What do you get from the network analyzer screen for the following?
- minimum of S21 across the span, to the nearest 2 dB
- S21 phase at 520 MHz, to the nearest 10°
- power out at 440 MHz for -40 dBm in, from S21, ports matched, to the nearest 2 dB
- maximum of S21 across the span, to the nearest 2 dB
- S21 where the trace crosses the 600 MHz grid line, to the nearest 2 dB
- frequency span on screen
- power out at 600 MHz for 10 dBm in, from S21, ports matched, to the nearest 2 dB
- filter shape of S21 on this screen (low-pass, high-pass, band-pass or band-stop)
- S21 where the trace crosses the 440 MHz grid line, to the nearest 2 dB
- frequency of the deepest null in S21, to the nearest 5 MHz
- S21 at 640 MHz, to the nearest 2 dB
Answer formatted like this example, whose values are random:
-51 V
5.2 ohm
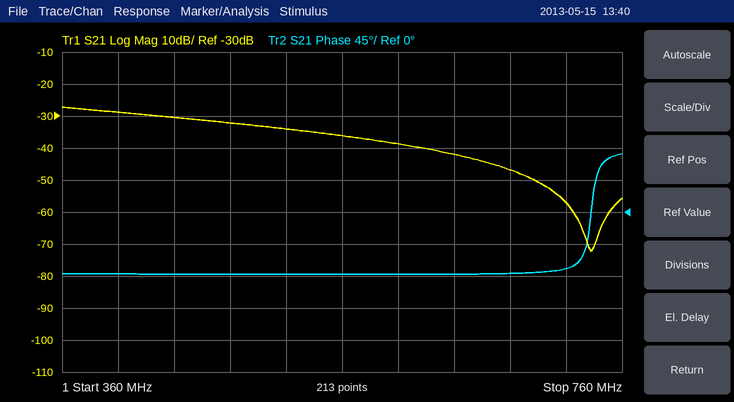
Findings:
-72 dB
-90°
-70 dBm
-28 dB
-38 dB
400 MHz
-28 dBm
low-pass
-30 dB
740 MHz
-42 dB
